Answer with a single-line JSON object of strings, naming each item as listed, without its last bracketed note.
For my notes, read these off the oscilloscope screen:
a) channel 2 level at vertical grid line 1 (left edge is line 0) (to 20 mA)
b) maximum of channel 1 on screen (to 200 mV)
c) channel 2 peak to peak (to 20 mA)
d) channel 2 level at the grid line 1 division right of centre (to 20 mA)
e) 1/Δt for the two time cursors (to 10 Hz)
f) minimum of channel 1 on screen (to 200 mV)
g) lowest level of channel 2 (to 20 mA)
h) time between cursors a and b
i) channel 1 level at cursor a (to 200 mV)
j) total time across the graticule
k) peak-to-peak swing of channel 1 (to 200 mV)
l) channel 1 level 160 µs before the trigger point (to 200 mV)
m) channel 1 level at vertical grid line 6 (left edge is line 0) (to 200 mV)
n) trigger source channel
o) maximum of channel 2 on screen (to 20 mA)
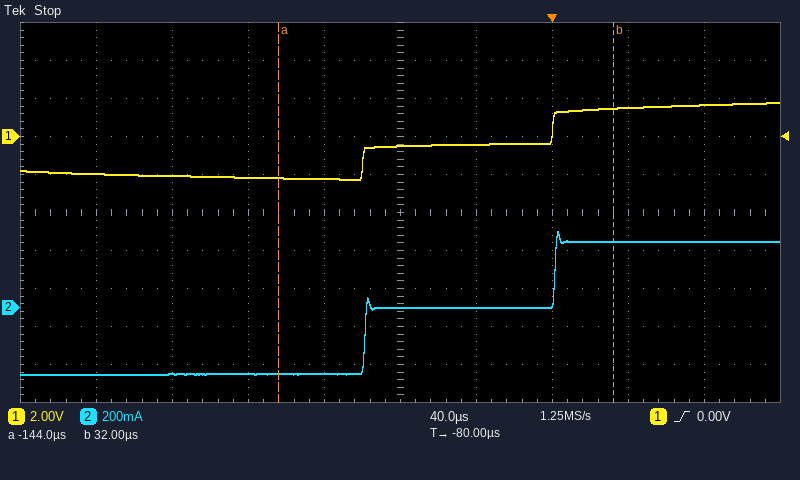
{"channel 2 level at vertical grid line 1 (left edge is line 0)": "-360 mA", "maximum of channel 1 on screen": "1.8 V", "channel 2 peak to peak": "760 mA", "channel 2 level at the grid line 1 division right of centre": "0 mA", "1/Δt for the two time cursors": "5.68 kHz", "minimum of channel 1 on screen": "-2.2 V", "lowest level of channel 2": "-360 mA", "time between cursors a and b": "176 µs", "channel 1 level at cursor a": "-2.2 V", "total time across the graticule": "400 µs", "peak-to-peak swing of channel 1": "4.0 V", "channel 1 level 160 µs before the trigger point": "-2.2 V", "channel 1 level at vertical grid line 6 (left edge is line 0)": "-400 mV", "trigger source channel": "channel 1", "maximum of channel 2 on screen": "400 mA"}
